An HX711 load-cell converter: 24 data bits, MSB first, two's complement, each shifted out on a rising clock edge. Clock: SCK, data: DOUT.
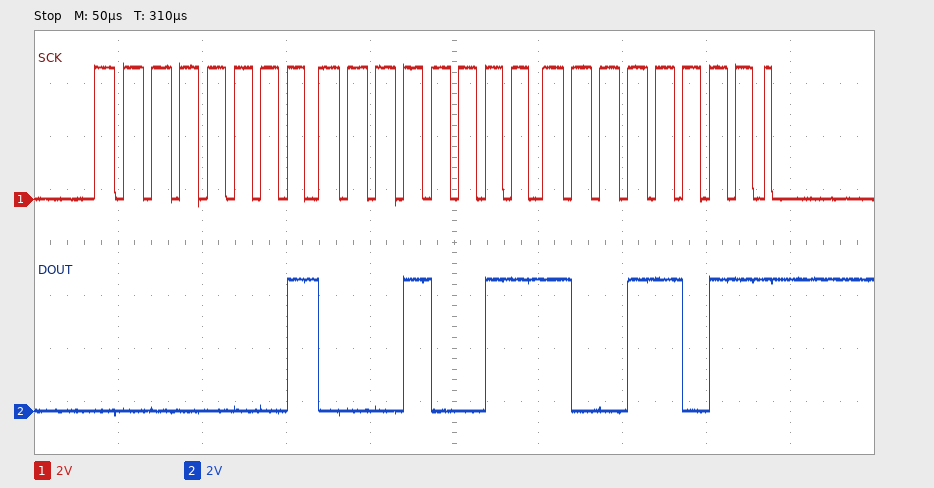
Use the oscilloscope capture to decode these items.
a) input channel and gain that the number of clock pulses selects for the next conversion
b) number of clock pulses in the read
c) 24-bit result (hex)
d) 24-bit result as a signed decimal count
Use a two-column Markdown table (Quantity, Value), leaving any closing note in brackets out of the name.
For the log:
| Quantity | Value |
|---|---|
| input channel and gain that the number of clock pulses selects for the next conversion | channel A, gain 128 |
| number of clock pulses in the read | 25 |
| 24-bit result | 0x01139B |
| 24-bit result as a signed decimal count | 70555 |
